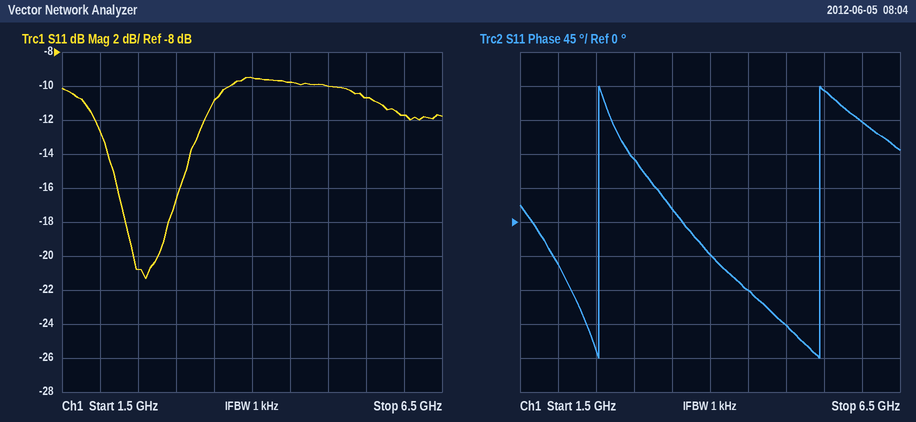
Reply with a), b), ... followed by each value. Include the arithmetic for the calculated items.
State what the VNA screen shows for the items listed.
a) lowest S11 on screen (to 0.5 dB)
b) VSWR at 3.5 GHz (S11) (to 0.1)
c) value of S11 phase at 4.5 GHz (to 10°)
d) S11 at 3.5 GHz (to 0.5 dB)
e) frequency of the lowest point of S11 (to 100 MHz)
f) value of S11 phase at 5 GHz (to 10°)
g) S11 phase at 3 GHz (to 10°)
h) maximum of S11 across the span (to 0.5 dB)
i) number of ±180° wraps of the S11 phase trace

a) -21.5 dB
b) |Γ| = 10^(-11/20) = 0.2818; VSWR = (1 + 0.2818)/(1 − 0.2818) ≈ 1.8
c) -90°
d) -11.0 dB
e) 2.6 GHz
f) -140°
g) 80°
h) -9.5 dB
i) 2
